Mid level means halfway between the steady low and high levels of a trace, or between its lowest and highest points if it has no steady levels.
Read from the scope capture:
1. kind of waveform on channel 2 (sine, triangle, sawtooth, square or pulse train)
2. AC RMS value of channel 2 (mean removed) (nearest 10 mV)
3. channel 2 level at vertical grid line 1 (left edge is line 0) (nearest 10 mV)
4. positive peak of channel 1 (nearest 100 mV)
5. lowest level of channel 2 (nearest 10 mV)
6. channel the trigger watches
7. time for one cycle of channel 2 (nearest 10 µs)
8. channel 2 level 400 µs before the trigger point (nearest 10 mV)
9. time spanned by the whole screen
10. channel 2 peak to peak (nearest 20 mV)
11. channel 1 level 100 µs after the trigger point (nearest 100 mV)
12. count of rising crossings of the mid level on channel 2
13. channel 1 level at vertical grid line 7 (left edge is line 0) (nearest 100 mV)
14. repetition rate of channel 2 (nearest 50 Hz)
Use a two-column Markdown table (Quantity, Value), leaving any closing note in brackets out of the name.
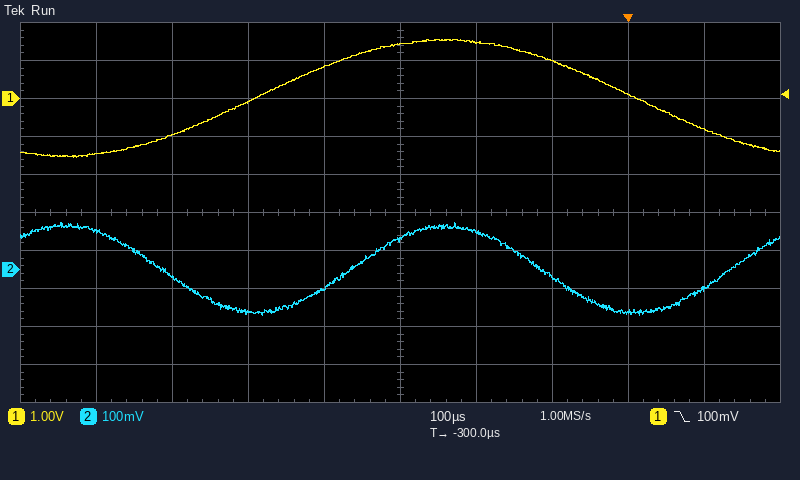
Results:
| Quantity | Value |
|---|---|
| kind of waveform on channel 2 | sine |
| AC RMS value of channel 2 (mean removed) | 80 mV |
| channel 2 level at vertical grid line 1 (left edge is line 0) | 100 mV |
| positive peak of channel 1 | 1.6 V |
| lowest level of channel 2 | -120 mV |
| channel the trigger watches | channel 1 |
| time for one cycle of channel 2 | 500 µs |
| channel 2 level 400 µs before the trigger point | -50 mV |
| time spanned by the whole screen | 1 ms |
| channel 2 peak to peak | 240 mV |
| channel 1 level 100 µs after the trigger point | -800 mV |
| count of rising crossings of the mid level on channel 2 | 2 |
| channel 1 level at vertical grid line 7 (left edge is line 0) | 1.0 V |
| repetition rate of channel 2 | 2.00 kHz |
